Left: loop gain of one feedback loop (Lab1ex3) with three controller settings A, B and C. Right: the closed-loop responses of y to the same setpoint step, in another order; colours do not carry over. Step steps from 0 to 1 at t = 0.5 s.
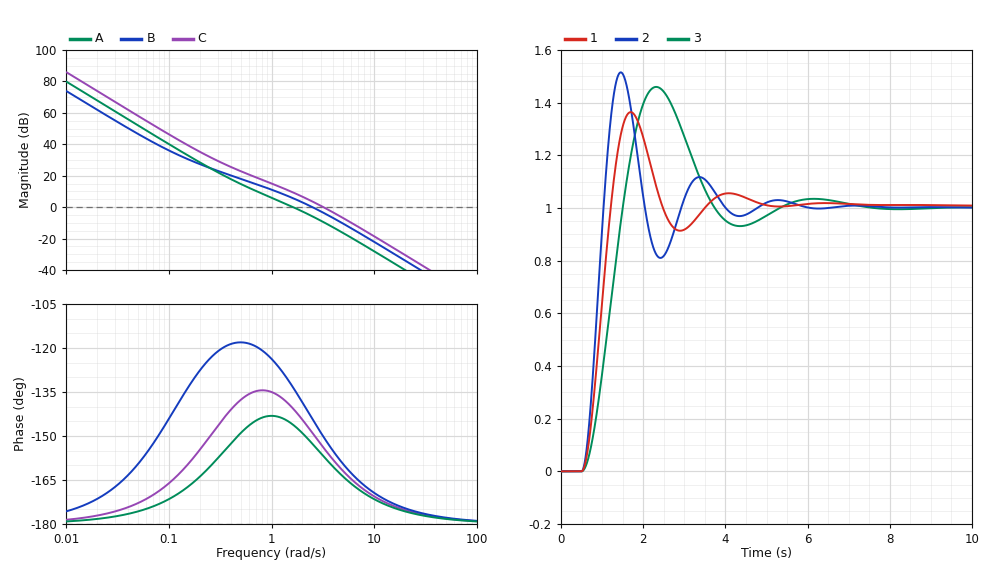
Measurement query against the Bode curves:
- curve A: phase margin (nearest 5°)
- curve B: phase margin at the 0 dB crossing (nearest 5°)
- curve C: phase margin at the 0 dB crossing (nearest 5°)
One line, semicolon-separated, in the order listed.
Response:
35°; 35°; 25°
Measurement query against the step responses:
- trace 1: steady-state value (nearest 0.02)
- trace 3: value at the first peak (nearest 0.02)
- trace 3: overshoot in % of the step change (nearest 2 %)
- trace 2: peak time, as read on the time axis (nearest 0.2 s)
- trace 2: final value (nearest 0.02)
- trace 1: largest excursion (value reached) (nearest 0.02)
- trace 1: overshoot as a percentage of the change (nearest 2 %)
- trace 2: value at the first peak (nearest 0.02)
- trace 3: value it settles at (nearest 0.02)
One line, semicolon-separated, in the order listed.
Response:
1.00; 1.46; 46 %; 1.4 s; 1.00; 1.36; 36 %; 1.52; 1.00
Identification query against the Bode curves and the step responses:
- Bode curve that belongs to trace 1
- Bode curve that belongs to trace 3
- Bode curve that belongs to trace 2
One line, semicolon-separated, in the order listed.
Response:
B; A; C
